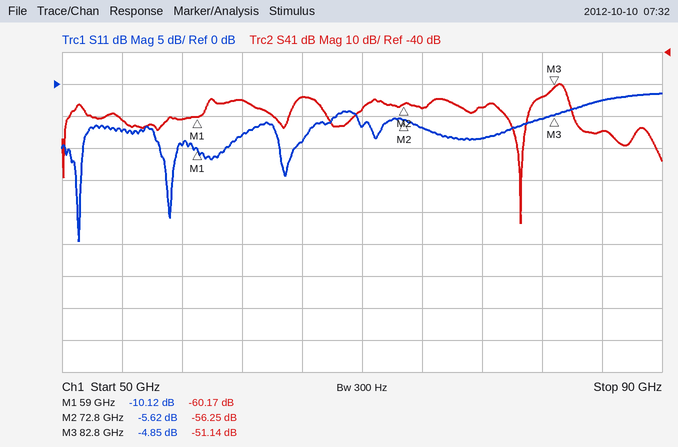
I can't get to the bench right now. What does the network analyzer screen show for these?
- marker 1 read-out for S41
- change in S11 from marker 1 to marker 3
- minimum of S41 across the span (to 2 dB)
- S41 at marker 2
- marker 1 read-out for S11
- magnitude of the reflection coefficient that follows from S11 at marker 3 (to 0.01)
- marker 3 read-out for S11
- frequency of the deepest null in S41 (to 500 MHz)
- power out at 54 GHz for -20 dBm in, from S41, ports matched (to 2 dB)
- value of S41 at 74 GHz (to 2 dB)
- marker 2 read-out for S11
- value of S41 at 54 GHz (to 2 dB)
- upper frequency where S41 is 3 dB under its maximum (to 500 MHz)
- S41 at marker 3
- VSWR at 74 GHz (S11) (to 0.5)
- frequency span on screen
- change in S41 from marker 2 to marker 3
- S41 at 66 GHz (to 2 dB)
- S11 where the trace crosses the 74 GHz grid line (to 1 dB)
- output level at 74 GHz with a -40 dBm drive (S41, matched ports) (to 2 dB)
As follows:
-60.17 dB
5.27 dB
-94 dB
-56.25 dB
-10.12 dB
0.57
-4.85 dB
80.5 GHz
-82 dBm
-58 dB
-5.62 dB
-62 dB
83.5 GHz
-51.14 dB
2.5
40 GHz
5.11 dB
-54 dB
-7 dB
-98 dBm
